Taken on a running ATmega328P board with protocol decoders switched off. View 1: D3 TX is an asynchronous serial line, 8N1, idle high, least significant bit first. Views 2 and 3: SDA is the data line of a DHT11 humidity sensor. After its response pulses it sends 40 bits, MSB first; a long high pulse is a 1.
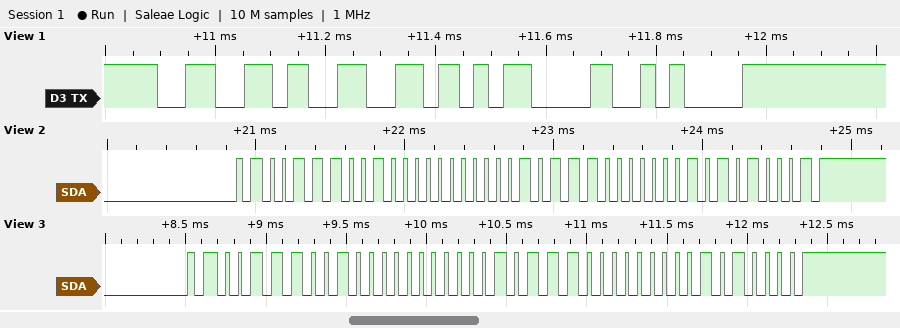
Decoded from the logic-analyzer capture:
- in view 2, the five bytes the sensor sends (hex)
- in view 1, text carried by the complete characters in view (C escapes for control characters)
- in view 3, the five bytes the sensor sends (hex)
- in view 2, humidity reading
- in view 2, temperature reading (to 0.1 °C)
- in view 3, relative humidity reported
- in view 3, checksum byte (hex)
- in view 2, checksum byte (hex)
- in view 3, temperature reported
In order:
39 00 17 01 51
"ff\r\n"
39 00 17 00 50
57 %
23.1 °C
57 %
0x50
0x51
23.0 °C
